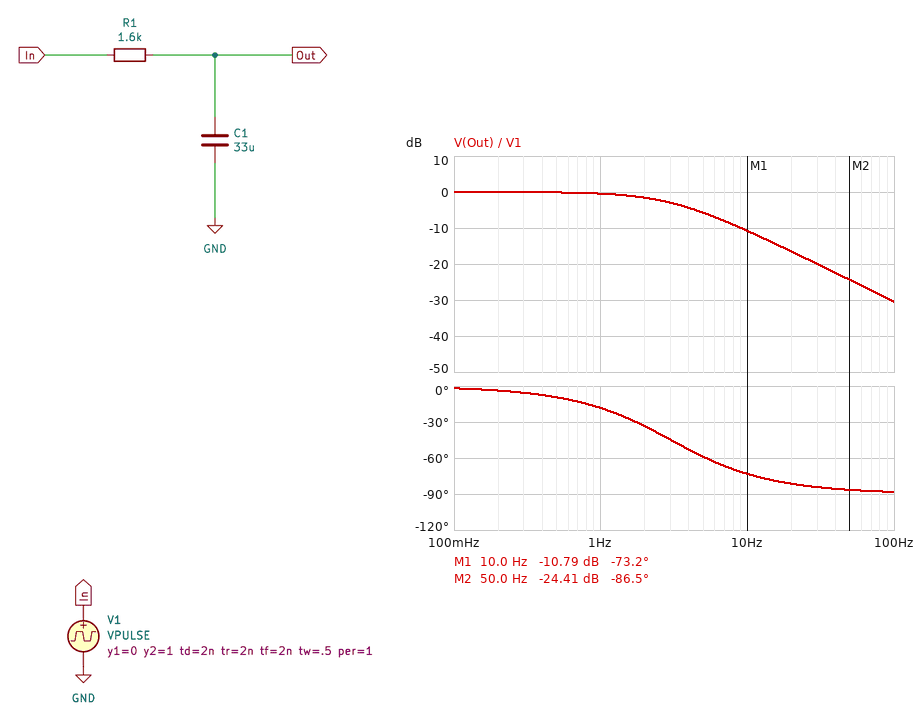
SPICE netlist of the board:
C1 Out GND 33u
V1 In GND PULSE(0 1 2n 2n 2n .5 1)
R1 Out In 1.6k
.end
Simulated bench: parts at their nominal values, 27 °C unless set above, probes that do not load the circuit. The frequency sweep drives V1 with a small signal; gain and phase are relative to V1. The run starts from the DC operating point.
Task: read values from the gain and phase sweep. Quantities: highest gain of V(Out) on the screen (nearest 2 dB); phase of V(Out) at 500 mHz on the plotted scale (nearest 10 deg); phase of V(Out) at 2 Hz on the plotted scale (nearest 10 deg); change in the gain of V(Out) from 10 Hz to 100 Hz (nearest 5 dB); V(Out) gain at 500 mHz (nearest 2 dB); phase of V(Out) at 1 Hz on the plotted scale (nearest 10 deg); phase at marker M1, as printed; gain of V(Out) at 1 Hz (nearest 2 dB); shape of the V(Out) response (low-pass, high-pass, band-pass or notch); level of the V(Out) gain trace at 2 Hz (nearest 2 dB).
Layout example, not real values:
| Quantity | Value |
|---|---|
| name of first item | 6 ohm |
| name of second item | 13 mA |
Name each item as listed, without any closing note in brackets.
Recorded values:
| Quantity | Value |
|---|---|
| highest gain of V(Out) on the screen | 0 dB |
| phase of V(Out) at 500 mHz on the plotted scale | -10 deg |
| phase of V(Out) at 2 Hz on the plotted scale | -30 deg |
| change in the gain of V(Out) from 10 Hz to 100 Hz | -20 dB |
| V(Out) gain at 500 mHz | 0 dB |
| phase of V(Out) at 1 Hz on the plotted scale | -20 deg |
| phase at marker M1, as printed | -73.2 deg |
| gain of V(Out) at 1 Hz | 0 dB |
| shape of the V(Out) response | low-pass |
| level of the V(Out) gain trace at 2 Hz | -2 dB |
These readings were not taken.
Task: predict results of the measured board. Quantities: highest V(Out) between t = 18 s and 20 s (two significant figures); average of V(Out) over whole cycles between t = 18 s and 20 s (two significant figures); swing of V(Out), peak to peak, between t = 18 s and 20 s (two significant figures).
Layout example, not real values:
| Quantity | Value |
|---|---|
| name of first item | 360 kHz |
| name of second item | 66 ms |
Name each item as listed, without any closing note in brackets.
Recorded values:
| Quantity | Value |
|---|---|
| highest V(Out) between t = 18 s and 20 s | 1.0 V |
| average of V(Out) over whole cycles between t = 18 s and 20 s | 500 mV |
| swing of V(Out), peak to peak, between t = 18 s and 20 s | 1.0 V |
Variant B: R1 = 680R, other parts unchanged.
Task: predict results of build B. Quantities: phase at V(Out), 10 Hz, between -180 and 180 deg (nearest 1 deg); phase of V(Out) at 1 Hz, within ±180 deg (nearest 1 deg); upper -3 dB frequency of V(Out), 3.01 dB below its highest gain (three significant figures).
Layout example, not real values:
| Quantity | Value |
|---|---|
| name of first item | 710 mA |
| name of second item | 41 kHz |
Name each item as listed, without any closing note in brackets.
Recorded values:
| Quantity | Value |
|---|---|
| phase at V(Out), 10 Hz, between -180 and 180 deg | -55 deg |
| phase of V(Out) at 1 Hz, within ±180 deg | -8 deg |
| upper -3 dB frequency of V(Out), 3.01 dB below its highest gain | 7.09 Hz |
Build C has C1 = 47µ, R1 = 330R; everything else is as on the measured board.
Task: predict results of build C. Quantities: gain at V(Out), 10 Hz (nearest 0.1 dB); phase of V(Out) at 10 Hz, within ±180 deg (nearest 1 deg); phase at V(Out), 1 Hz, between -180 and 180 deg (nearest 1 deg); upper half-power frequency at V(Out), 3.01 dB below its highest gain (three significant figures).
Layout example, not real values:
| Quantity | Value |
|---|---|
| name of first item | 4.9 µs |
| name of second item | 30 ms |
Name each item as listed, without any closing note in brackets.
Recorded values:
| Quantity | Value |
|---|---|
| gain at V(Out), 10 Hz | -2.9 dB |
| phase of V(Out) at 10 Hz, within ±180 deg | -44 deg |
| phase at V(Out), 1 Hz, between -180 and 180 deg | -6 deg |
| upper half-power frequency at V(Out), 3.01 dB below its highest gain | 10.3 Hz |
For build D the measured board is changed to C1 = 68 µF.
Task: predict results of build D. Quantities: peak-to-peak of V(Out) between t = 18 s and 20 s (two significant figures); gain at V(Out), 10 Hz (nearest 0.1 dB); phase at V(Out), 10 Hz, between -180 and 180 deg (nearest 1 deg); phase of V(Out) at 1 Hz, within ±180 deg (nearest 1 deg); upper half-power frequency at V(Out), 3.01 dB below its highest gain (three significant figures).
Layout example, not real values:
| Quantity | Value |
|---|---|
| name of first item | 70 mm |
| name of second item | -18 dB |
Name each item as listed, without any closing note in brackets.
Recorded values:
| Quantity | Value |
|---|---|
| peak-to-peak of V(Out) between t = 18 s and 20 s | 980 mV |
| gain at V(Out), 10 Hz | -16.8 dB |
| phase at V(Out), 10 Hz, between -180 and 180 deg | -82 deg |
| phase of V(Out) at 1 Hz, within ±180 deg | -34 deg |
| upper half-power frequency at V(Out), 3.01 dB below its highest gain | 1.46 Hz |
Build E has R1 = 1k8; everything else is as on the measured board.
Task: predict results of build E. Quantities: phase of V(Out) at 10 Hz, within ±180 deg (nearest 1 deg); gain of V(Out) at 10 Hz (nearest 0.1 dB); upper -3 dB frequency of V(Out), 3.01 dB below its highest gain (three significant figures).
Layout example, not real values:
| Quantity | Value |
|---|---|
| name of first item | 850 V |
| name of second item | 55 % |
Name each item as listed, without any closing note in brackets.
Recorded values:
| Quantity | Value |
|---|---|
| phase of V(Out) at 10 Hz, within ±180 deg | -75 deg |
| gain of V(Out) at 10 Hz | -11.7 dB |
| upper -3 dB frequency of V(Out), 3.01 dB below its highest gain | 2.68 Hz |
